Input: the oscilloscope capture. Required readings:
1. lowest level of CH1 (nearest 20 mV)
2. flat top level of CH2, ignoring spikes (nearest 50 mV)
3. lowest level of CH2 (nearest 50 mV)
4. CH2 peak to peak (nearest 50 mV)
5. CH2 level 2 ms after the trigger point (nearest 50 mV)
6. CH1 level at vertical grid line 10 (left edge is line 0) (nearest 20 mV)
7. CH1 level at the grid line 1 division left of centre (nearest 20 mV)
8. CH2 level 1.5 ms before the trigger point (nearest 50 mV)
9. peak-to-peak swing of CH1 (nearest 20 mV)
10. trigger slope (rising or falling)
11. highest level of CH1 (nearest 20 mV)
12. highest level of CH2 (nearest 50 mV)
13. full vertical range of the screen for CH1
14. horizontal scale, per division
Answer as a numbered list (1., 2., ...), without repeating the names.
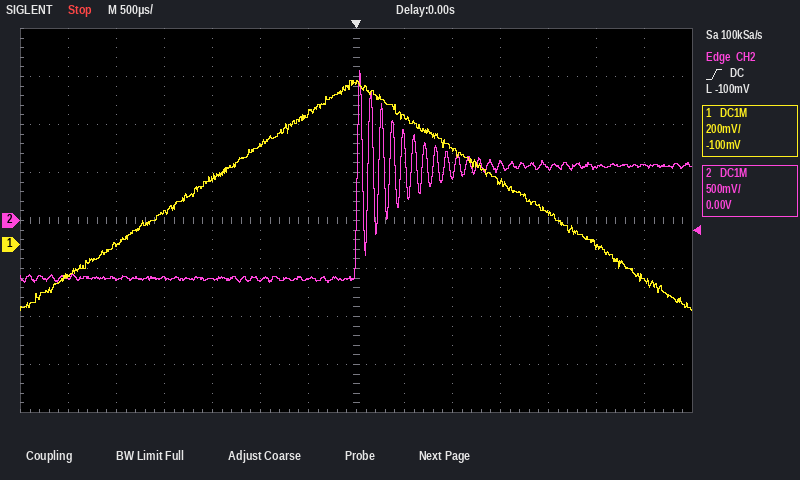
1. -280 mV
2. 550 mV
3. -650 mV
4. 2.20 V
5. 550 mV
6. 260 mV
7. 540 mV
8. -600 mV
9. 960 mV
10. rising
11. 680 mV
12. 1.55 V
13. 1.6 V
14. 500 µs
